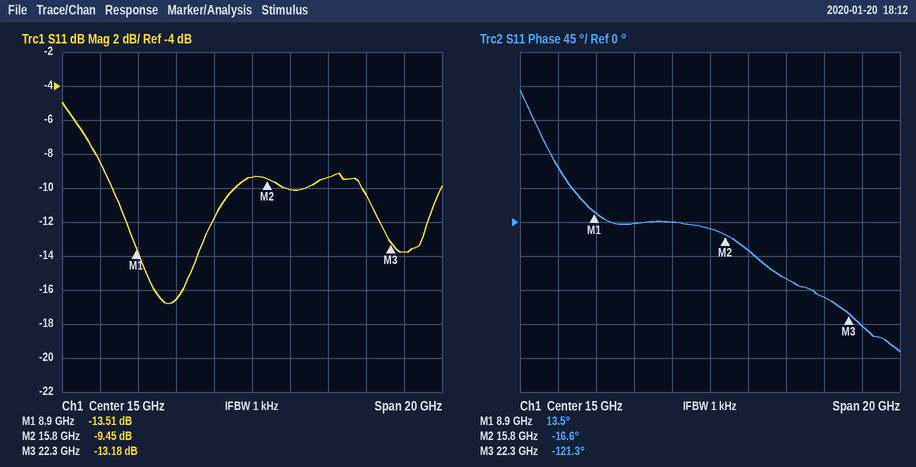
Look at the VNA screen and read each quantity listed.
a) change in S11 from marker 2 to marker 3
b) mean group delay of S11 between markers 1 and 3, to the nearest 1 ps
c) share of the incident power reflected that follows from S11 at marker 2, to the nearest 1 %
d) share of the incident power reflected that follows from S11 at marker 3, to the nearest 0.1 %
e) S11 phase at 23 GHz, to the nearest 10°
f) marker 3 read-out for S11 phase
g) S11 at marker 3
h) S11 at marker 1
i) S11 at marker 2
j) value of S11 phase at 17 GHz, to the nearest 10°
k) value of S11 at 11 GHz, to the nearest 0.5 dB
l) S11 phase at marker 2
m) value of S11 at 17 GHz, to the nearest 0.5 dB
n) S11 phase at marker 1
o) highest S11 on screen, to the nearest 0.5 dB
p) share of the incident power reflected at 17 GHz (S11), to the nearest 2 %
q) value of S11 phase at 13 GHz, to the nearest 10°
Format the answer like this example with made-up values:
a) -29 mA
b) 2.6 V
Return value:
a) -3.73 dB
b) 28 ps
c) 11 %
d) 4.8 %
e) -140°
f) -121.3°
g) -13.18 dB
h) -13.51 dB
i) -9.45 dB
j) -40°
k) -16.5 dB
l) -16.6°
m) -10.0 dB
n) 13.5°
o) -5.0 dB
p) 10 %
q) 0°
